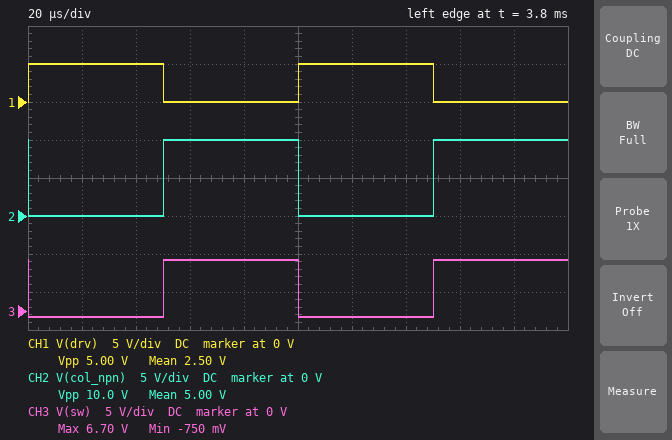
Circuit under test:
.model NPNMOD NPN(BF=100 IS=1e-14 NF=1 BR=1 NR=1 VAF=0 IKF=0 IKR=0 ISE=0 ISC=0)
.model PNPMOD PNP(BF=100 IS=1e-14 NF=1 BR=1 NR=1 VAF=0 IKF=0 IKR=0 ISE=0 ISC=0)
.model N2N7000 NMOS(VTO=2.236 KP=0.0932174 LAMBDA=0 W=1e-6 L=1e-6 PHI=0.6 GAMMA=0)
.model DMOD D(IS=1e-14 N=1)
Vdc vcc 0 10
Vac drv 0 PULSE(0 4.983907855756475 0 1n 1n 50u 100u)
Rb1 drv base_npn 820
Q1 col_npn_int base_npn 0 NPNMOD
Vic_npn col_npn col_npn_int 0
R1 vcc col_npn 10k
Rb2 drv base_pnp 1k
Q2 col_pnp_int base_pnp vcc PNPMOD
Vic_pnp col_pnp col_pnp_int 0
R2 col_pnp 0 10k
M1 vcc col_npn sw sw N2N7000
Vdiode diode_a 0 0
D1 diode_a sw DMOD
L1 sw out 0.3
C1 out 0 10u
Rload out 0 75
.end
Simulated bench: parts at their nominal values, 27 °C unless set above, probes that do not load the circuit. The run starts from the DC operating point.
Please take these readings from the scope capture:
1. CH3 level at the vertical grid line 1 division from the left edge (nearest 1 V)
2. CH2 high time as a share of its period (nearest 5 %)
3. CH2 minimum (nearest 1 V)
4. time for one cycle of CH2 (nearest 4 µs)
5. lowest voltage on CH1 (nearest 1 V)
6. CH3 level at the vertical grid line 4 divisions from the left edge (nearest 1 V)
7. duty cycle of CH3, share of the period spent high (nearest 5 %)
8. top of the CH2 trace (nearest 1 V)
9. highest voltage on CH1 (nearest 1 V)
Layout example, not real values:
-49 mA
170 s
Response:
-1 V
50 %
0 V
100 µs
0 V
7 V
50 %
10 V
5 V
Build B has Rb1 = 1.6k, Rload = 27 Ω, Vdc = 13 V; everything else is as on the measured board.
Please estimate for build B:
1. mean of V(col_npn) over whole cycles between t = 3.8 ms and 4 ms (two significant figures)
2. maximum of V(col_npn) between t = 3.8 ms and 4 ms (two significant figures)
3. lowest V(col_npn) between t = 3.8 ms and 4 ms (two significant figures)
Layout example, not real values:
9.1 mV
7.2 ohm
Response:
6.5 V
13 V
24 mV
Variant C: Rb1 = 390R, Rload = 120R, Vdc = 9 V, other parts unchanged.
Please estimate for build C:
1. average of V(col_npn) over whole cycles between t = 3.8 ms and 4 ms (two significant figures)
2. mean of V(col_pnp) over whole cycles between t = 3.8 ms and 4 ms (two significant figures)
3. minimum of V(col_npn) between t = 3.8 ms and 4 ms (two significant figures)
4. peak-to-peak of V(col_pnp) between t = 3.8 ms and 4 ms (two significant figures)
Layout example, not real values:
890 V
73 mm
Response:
4.5 V
9.0 V
19 mV
2.0 mV
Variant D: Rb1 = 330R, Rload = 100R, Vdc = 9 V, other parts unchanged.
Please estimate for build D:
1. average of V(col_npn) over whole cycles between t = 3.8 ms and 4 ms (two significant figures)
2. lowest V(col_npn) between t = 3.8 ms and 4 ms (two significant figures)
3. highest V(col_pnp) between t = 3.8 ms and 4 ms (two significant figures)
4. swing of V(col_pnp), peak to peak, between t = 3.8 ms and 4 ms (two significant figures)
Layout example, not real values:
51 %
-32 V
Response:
4.5 V
19 mV
9.0 V
2.0 mV
